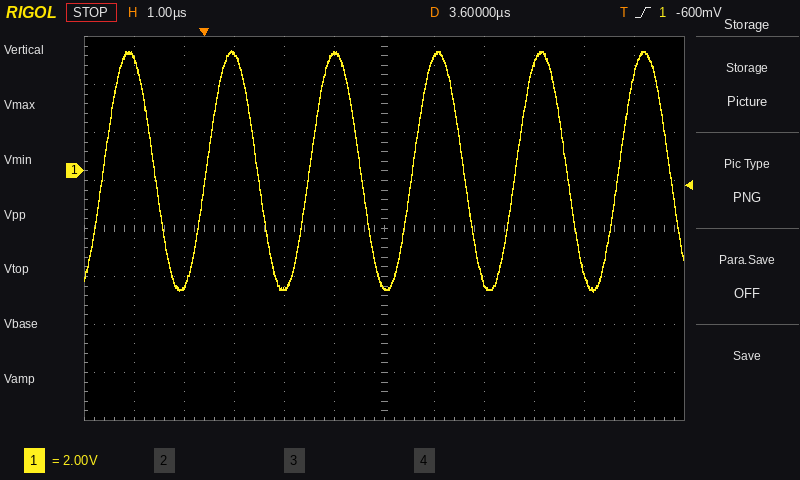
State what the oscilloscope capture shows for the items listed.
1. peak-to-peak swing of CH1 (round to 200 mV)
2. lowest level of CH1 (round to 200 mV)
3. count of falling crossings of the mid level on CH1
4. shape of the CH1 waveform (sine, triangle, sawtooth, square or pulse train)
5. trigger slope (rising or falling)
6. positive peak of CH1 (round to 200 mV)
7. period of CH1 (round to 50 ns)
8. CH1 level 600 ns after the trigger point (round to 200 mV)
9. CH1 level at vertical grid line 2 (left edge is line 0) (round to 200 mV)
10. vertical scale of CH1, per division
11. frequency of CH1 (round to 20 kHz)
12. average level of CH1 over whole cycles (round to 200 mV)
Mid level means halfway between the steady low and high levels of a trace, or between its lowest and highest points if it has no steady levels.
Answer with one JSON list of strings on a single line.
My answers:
["10.0 V", "-5.0 V", "6", "sine", "rising", "5.0 V", "2.05 µs", "4.8 V", "-4.8 V", "2 V", "480 kHz", "0.0 V"]
